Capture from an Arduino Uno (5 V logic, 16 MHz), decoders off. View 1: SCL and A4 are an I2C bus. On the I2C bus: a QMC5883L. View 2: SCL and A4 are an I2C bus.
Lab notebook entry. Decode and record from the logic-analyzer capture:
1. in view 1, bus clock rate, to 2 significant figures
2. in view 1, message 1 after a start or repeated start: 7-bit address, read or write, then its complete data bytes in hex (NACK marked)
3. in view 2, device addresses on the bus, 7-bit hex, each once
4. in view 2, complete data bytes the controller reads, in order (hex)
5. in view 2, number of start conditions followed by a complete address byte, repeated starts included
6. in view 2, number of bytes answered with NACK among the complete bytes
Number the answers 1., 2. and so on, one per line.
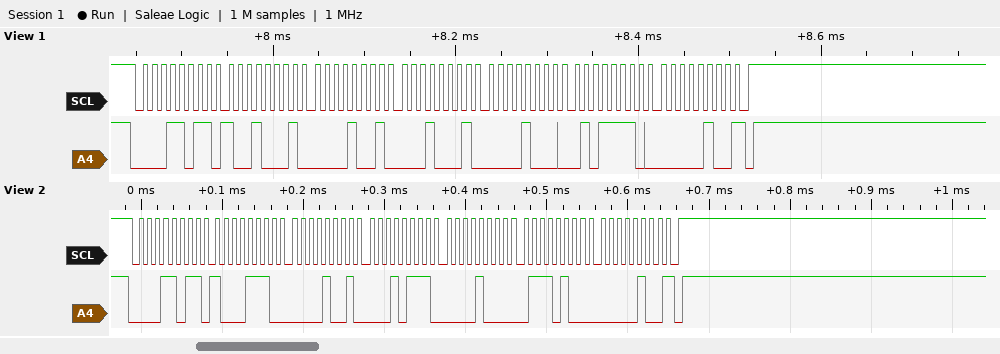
1. 100 kHz
2. 0x0D read: 91 09 11 08 5E 04 NACK
3. 0x0D
4. 8E 09 17 08 74 04
5. 1
6. 1
